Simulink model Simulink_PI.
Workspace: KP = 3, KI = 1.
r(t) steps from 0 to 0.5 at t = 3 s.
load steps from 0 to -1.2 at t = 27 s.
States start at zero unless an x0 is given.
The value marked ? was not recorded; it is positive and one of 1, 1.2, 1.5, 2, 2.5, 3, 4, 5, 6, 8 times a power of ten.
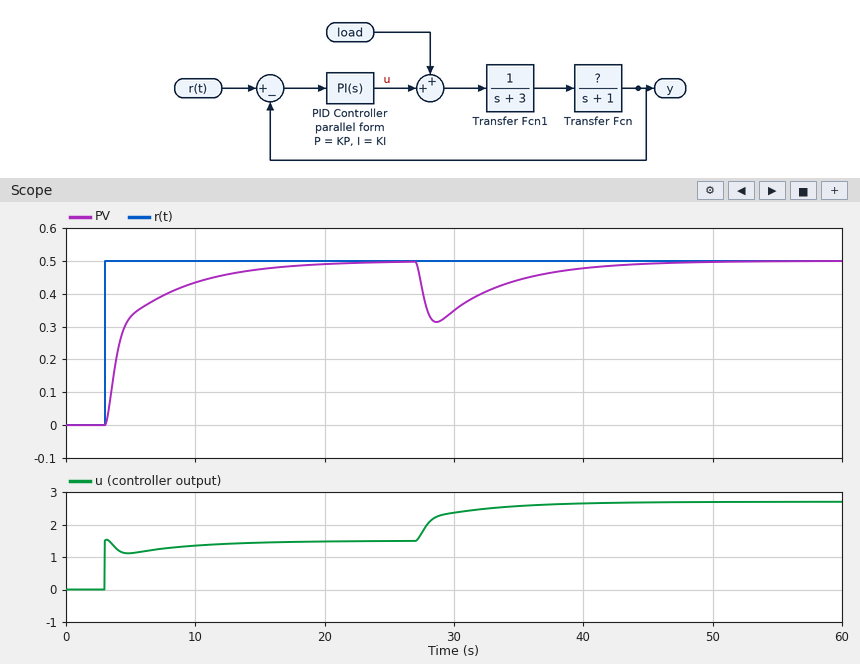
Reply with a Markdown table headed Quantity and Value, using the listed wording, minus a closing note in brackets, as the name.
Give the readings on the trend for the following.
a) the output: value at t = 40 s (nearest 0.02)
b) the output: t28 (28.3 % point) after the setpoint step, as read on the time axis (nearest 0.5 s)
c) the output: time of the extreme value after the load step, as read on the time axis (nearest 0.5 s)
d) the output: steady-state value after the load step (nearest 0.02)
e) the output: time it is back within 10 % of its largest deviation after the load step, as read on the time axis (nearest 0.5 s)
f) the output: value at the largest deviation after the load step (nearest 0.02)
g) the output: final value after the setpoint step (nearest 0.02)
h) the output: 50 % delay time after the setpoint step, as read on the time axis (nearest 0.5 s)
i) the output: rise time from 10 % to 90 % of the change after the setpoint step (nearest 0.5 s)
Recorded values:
| Quantity | Value |
|---|---|
| the output: value at t = 40 s | 0.48 |
| the output: t28 (28.3 % point) after the setpoint step, as read on the time axis | 3.5 s |
| the output: time of the extreme value after the load step, as read on the time axis | 28.5 s |
| the output: steady-state value after the load step | 0.50 |
| the output: time it is back within 10 % of its largest deviation after the load step, as read on the time axis | 41.0 s |
| the output: value at the largest deviation after the load step | 0.32 |
| the output: final value after the setpoint step | 0.50 |
| the output: 50 % delay time after the setpoint step, as read on the time axis | 4.0 s |
| the output: rise time from 10 % to 90 % of the change after the setpoint step | 8.0 s |
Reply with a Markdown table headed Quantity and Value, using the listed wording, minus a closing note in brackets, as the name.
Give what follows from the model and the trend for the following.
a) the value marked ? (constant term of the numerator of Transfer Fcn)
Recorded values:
| Quantity | Value |
|---|---|
| the value marked ? | 1 |
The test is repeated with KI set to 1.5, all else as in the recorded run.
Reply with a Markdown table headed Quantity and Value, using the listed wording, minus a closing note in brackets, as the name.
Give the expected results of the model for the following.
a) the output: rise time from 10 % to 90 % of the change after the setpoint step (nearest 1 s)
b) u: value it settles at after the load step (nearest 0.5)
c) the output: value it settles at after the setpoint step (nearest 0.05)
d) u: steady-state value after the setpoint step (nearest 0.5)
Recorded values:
| Quantity | Value |
|---|---|
| the output: rise time from 10 % to 90 % of the change after the setpoint step | 5 s |
| u: value it settles at after the load step | 2.5 |
| the output: value it settles at after the setpoint step | 0.50 |
| u: steady-state value after the setpoint step | 1.5 |
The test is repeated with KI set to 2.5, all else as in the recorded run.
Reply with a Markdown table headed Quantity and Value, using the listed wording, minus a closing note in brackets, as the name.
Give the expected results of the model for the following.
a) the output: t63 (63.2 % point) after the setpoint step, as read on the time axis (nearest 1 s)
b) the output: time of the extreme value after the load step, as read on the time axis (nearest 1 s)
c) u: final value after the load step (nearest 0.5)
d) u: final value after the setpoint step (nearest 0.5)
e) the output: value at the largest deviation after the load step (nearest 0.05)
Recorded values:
| Quantity | Value |
|---|---|
| the output: t63 (63.2 % point) after the setpoint step, as read on the time axis | 4 s |
| the output: time of the extreme value after the load step, as read on the time axis | 28 s |
| u: final value after the load step | 2.5 |
| u: final value after the setpoint step | 1.5 |
| the output: value at the largest deviation after the load step | 0.35 |
